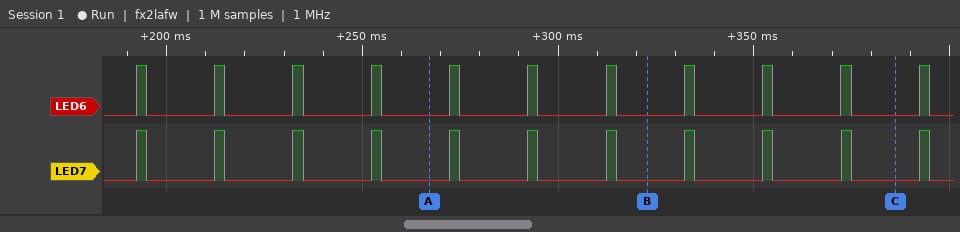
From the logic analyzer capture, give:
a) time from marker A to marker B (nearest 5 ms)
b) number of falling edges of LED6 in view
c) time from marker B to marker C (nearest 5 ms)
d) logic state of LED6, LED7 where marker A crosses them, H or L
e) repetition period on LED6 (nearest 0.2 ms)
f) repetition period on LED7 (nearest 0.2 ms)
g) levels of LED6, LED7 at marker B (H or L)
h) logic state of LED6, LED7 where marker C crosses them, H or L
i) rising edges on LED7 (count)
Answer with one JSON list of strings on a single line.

["55 ms", "11", "65 ms", "LED6=L, LED7=L", "20 ms", "20 ms", "LED6=L, LED7=L", "LED6=L, LED7=L", "11"]
